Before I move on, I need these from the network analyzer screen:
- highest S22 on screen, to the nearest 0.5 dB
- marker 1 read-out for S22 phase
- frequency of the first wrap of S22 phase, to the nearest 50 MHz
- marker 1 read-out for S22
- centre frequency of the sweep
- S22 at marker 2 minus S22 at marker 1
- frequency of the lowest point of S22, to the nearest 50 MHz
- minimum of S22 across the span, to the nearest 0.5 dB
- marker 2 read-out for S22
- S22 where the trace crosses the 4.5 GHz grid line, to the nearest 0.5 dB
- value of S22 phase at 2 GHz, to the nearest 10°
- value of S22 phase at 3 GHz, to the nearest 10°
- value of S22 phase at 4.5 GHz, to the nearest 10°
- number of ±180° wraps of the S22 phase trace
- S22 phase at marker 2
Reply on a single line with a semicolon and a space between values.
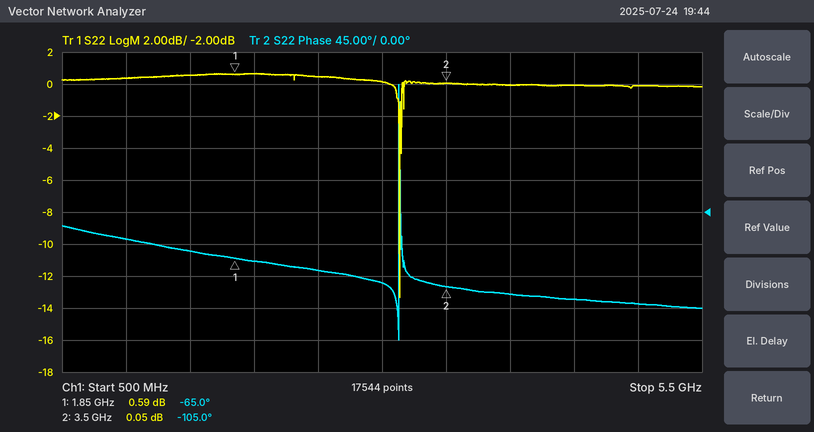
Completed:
0.5 dB; -65.0°; 3.15 GHz; 0.59 dB; 3 GHz; -0.54 dB; 3.15 GHz; -13.5 dB; 0.05 dB; 0.0 dB; -70°; -100°; -120°; 1; -105.0°
